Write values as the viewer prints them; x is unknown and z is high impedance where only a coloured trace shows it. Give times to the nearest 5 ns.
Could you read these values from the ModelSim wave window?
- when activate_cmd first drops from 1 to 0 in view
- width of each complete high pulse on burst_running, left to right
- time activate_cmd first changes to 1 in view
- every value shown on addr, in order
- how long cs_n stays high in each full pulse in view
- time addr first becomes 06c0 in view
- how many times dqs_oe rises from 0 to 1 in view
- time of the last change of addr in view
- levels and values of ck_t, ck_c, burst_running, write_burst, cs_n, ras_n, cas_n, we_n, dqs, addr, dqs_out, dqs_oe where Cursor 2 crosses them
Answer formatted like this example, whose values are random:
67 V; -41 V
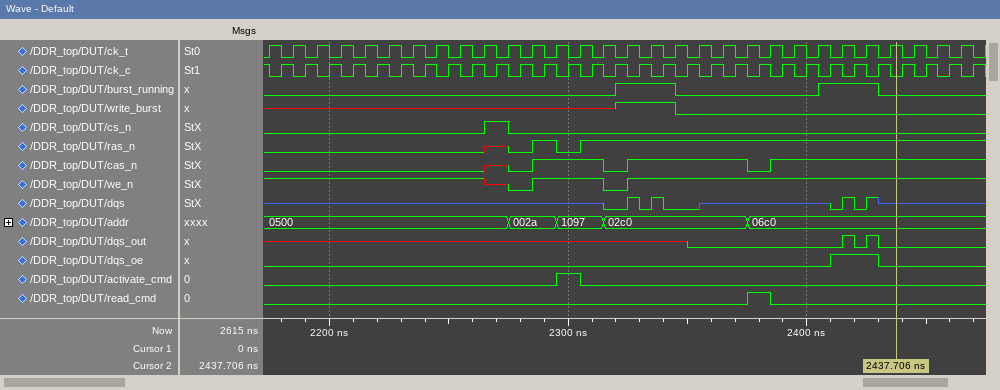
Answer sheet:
2305 ns; 25 ns, 25 ns; 2295 ns; 0500, 002a, 1097, 02c0, 06c0; 10 ns; 2375 ns; 1; 2375 ns; ck_t=1, ck_c=0, burst_running=0, write_burst=0, cs_n=0, ras_n=1, cas_n=1, we_n=1, dqs=z, addr=06c0, dqs_out=0, dqs_oe=0
